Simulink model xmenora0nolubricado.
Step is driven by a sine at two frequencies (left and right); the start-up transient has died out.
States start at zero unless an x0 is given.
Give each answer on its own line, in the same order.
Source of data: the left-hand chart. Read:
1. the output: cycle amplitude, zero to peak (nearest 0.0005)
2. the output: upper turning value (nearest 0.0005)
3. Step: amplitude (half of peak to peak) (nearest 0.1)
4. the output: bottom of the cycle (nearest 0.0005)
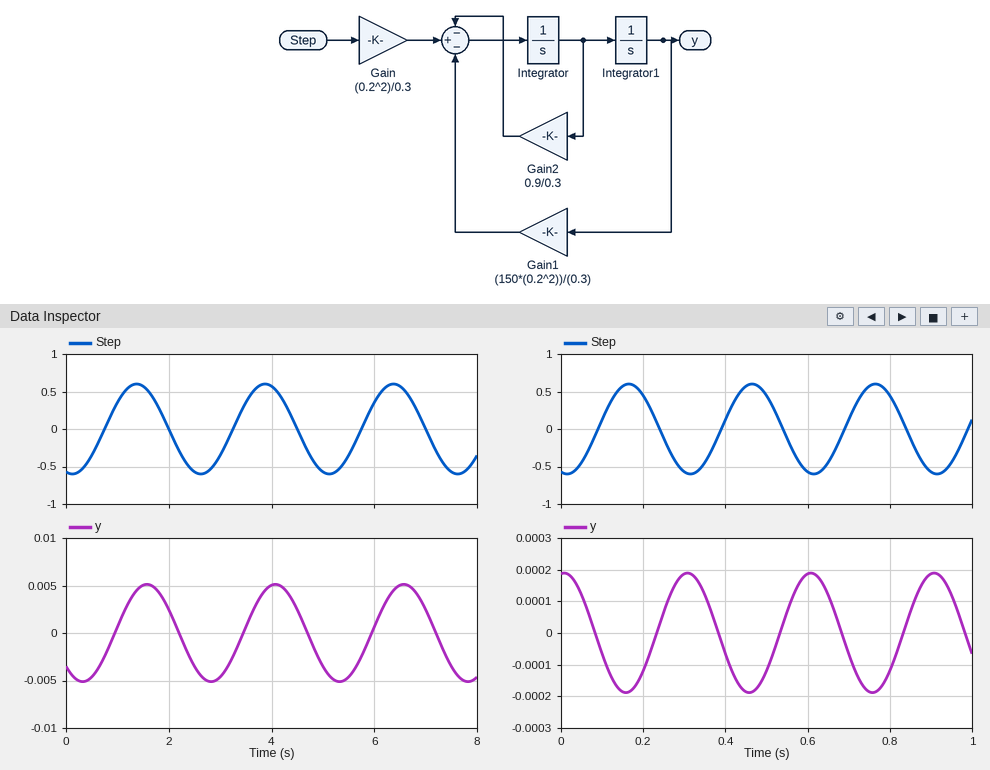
0.0050
0.0050
0.6
-0.0050
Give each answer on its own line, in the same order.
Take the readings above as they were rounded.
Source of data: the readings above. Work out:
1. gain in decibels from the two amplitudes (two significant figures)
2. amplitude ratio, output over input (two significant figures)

-42 dB
0.0083
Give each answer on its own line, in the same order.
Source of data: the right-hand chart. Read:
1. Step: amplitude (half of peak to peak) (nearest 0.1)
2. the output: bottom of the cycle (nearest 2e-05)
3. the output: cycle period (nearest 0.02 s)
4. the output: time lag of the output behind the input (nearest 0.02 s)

0.6
-0.00018
0.30 s
0.14 s
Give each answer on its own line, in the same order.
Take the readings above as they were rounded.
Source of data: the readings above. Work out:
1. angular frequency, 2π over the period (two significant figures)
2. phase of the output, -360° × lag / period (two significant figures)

21 rad/s
-170°
